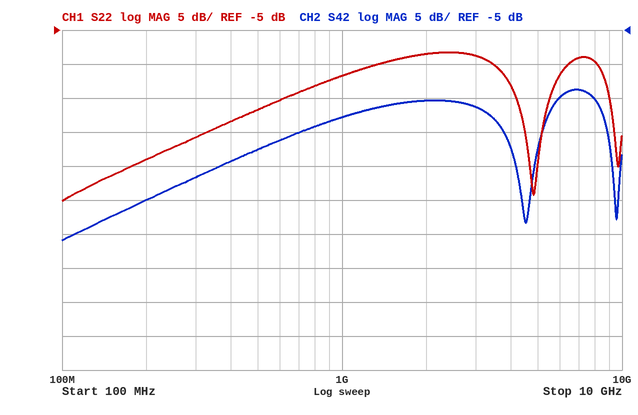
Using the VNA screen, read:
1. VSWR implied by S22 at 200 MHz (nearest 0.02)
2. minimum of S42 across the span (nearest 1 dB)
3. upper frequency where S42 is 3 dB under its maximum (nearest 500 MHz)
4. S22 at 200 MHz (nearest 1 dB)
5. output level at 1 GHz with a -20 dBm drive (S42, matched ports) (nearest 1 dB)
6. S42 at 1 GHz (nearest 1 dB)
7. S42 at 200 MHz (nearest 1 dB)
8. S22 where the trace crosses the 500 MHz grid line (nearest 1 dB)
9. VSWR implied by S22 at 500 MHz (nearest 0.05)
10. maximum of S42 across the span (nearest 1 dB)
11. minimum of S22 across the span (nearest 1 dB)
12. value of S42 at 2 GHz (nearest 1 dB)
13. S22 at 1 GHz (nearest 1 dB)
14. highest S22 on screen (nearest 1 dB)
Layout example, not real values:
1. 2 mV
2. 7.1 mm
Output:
1. 1.14
2. -36 dB
3. 8.5 GHz
4. -24 dB
5. -38 dBm
6. -18 dB
7. -30 dB
8. -17 dB
9. 1.35
10. -14 dB
11. -30 dB
12. -15 dB
13. -12 dB
14. -8 dB
